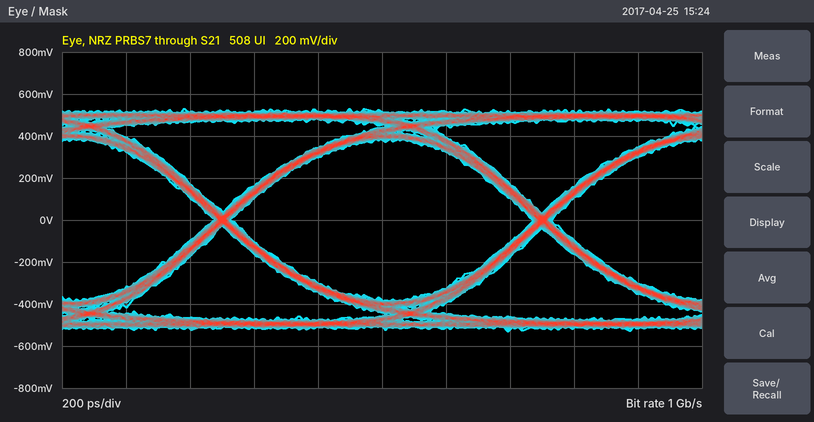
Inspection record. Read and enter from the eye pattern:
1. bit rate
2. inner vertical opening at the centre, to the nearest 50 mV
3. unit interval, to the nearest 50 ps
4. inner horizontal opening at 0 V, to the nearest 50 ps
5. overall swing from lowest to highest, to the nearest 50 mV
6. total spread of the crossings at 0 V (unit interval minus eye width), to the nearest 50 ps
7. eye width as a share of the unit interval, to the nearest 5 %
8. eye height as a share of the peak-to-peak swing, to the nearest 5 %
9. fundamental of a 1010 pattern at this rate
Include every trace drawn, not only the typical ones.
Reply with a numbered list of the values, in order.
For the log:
1. 1 Gb/s
2. 750 mV
3. 1.00 ns
4. 950 ps
5. 1.05 V
6. 50 ps
7. 95 %
8. 70 %
9. 500 MHz
